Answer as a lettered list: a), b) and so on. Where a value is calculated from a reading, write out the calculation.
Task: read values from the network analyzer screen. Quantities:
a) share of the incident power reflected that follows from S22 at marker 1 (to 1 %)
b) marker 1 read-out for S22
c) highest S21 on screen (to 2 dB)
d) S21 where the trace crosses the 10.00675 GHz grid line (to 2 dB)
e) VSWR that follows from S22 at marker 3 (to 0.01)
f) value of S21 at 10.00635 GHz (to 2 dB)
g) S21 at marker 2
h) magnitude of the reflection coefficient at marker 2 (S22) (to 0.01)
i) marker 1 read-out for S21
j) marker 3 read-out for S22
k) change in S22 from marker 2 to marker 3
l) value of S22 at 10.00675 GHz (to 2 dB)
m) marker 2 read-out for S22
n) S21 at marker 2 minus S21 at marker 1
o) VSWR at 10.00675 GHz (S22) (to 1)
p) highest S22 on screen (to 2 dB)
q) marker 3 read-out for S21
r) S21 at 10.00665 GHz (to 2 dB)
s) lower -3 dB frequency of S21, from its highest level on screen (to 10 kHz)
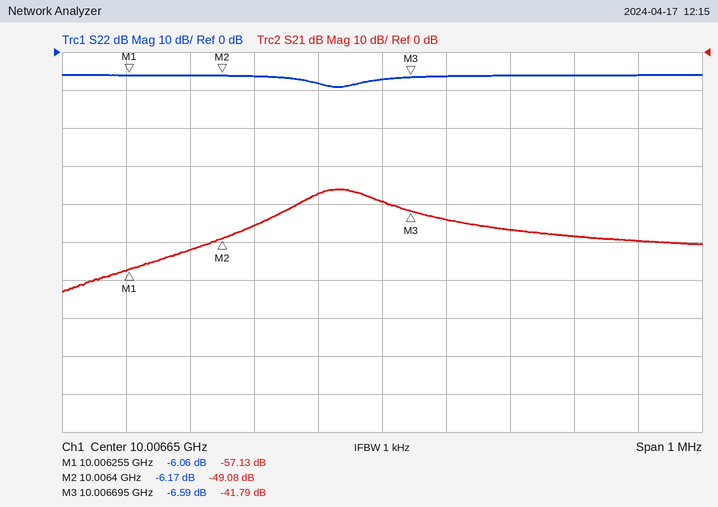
a) 10^(-6.06/10) ≈ 25 %
b) -6.06 dB
c) -36 dB
d) -44 dB
e) (1 + 0.4683)/(1 − 0.4683) ≈ 2.76
f) -52 dB
g) -49.08 dB
h) 10^(-6.17/20) ≈ 0.49
i) -57.13 dB
j) -6.59 dB
k) -6.59 − (-6.17) = -0.42 dB
l) -6 dB
m) -6.17 dB
n) -49.08 − (-57.13) = 8.05 dB
o) |Γ| = 10^(-6/20) = 0.5012; VSWR = (1 + 0.5012)/(1 − 0.5012) ≈ 3
p) -6 dB
q) -41.79 dB
r) -40 dB
s) 10.00653 GHz
